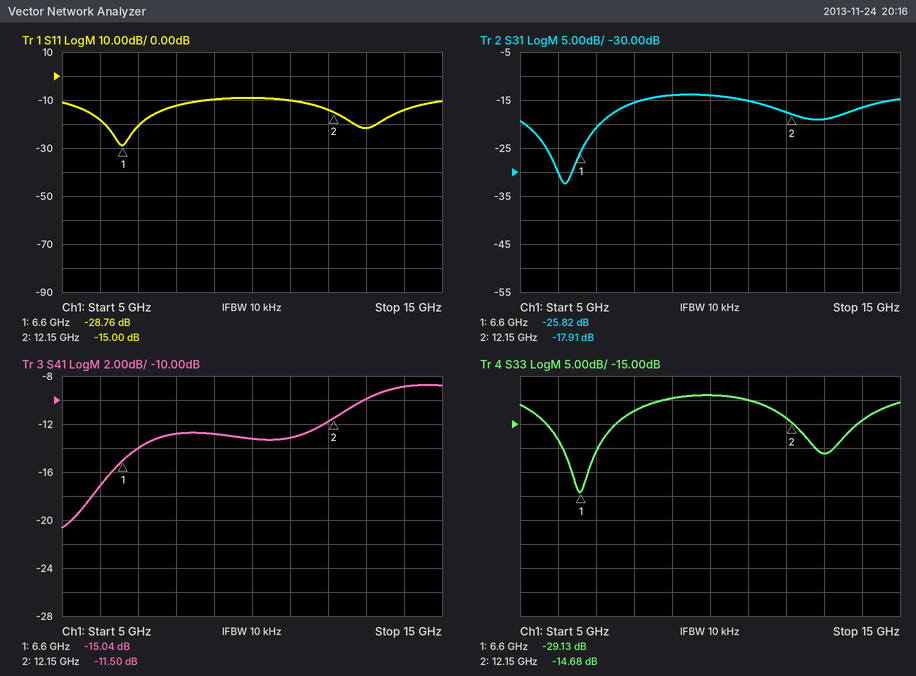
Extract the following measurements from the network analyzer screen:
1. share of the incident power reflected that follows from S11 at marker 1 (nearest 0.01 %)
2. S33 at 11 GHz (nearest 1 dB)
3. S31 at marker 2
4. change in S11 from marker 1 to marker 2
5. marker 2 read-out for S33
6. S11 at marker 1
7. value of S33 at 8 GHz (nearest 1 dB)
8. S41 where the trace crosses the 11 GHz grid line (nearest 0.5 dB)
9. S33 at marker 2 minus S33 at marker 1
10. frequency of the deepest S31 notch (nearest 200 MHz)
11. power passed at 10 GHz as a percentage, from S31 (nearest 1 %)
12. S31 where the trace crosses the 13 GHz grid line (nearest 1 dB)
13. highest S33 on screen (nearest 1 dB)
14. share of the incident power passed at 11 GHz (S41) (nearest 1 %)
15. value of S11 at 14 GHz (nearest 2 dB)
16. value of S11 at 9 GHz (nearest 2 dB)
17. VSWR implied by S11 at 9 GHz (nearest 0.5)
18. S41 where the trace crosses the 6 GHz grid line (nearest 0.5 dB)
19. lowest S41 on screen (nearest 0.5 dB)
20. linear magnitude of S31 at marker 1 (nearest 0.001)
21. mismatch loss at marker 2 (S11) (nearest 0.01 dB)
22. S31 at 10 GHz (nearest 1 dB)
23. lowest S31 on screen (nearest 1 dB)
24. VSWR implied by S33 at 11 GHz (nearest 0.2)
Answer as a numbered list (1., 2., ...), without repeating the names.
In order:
1. 0.13 %
2. -10 dB
3. -17.91 dB
4. 13.76 dB
5. -14.68 dB
6. -28.76 dB
7. -12 dB
8. -13.0 dB
9. 14.45 dB
10. 6.2 GHz
11. 4 %
12. -19 dB
13. -9 dB
14. 5 %
15. -14 dB
16. -10 dB
17. 2.0
18. -17.0 dB
19. -20.5 dB
20. 0.051
21. 0.14 dB
22. -14 dB
23. -32 dB
24. 2.0
